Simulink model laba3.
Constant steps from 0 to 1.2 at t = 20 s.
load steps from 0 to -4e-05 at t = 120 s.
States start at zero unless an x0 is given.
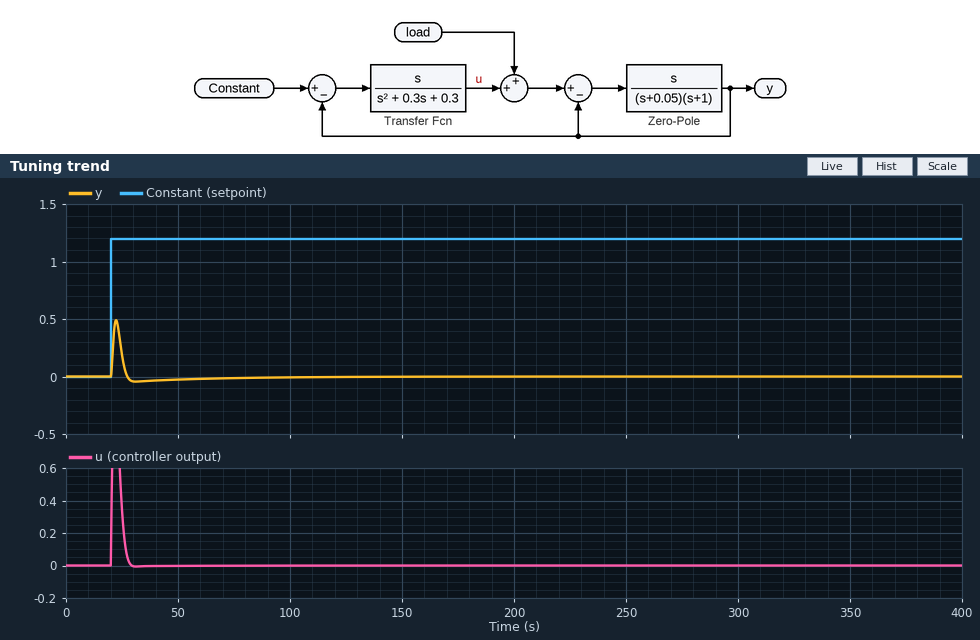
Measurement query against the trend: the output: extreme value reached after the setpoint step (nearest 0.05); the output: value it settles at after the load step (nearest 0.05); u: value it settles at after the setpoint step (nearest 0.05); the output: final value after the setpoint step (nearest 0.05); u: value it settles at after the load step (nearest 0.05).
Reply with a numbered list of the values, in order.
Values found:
1. 0.50
2. 0.00
3. 0.00
4. 0.00
5. 0.00
